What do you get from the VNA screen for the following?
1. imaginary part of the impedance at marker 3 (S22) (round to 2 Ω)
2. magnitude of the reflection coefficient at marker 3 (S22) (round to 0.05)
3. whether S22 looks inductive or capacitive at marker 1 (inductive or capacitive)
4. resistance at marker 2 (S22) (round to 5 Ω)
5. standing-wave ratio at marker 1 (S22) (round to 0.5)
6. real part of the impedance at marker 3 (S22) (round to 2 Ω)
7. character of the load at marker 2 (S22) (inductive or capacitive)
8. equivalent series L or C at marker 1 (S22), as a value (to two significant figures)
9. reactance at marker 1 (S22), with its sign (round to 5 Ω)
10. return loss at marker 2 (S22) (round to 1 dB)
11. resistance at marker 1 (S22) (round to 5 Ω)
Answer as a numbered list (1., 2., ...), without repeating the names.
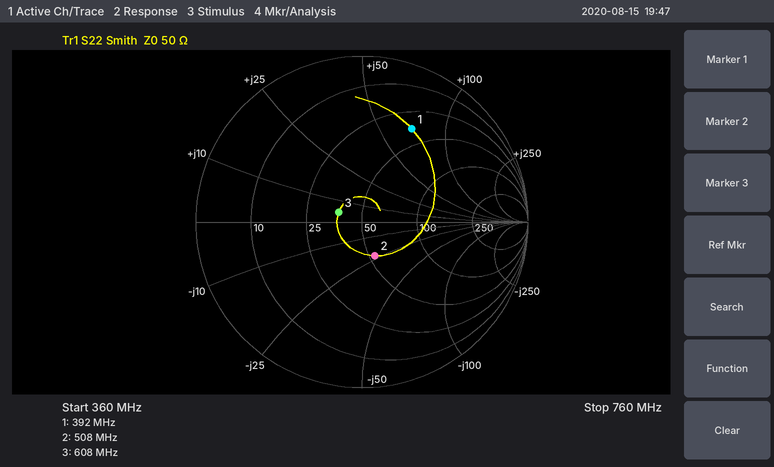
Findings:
1. +4 Ω
2. 0.15
3. inductive
4. 55 Ω
5. 4.5
6. 38 Ω
7. capacitive
8. 28 nH
9. +70 Ω
10. 13 dB
11. 35 Ω
